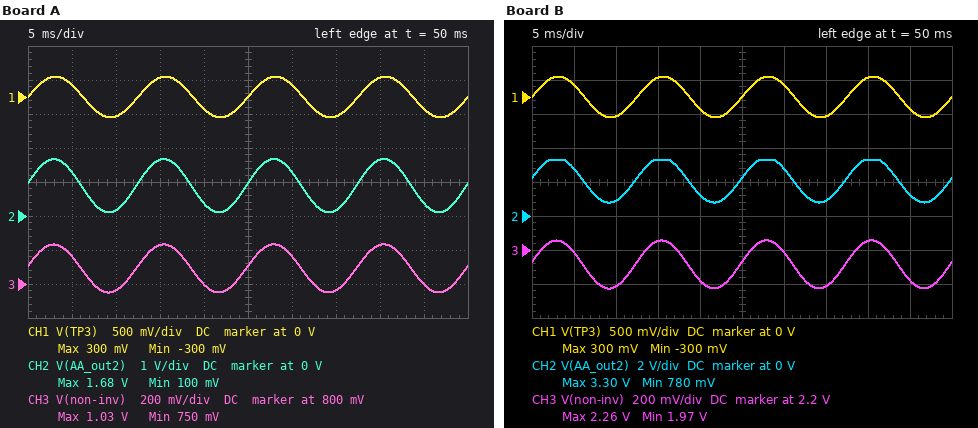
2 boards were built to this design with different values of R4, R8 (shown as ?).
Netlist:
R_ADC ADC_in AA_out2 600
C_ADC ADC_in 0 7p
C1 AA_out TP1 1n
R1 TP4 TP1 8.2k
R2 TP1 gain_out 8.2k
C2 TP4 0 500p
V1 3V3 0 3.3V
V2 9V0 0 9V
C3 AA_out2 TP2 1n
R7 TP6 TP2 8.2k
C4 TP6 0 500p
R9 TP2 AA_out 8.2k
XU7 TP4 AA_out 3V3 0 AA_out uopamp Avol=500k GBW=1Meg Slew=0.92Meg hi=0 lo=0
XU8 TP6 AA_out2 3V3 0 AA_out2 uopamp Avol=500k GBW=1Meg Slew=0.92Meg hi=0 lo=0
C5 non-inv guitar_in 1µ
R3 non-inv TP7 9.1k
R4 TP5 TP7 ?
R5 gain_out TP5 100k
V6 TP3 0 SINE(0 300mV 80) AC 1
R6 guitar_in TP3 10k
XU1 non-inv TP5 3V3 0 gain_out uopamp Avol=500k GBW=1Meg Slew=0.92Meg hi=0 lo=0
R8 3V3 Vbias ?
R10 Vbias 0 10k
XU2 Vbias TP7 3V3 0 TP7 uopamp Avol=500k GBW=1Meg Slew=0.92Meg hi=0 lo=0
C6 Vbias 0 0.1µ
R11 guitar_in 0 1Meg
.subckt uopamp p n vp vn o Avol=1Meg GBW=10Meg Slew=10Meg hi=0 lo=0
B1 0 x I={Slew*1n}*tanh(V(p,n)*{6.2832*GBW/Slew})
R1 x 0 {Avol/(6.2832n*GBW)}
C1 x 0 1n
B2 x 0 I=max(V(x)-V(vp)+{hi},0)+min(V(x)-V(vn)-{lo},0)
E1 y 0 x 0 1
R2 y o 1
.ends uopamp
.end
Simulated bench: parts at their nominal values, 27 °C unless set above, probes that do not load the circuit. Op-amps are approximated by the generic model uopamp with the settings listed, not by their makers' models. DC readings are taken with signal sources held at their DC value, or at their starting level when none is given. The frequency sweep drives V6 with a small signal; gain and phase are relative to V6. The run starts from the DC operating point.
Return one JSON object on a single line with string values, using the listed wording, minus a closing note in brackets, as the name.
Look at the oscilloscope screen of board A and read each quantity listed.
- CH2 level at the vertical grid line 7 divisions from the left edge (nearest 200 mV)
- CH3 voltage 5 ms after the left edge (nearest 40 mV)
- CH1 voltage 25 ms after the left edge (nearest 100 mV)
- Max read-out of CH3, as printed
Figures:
{"CH2 level at the vertical grid line 7 divisions from the left edge": "200 mV", "CH3 voltage 5 ms after the left edge": "960 mV", "CH1 voltage 25 ms after the left edge": "0 V", "Max read-out of CH3, as printed": "1.03 V"}
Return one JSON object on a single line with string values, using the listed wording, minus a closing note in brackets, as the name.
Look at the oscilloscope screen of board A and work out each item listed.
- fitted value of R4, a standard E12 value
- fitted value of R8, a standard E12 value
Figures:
{"fitted value of R4, a standard E12 value": "22 kΩ", "fitted value of R8, a standard E12 value": "27 kΩ"}
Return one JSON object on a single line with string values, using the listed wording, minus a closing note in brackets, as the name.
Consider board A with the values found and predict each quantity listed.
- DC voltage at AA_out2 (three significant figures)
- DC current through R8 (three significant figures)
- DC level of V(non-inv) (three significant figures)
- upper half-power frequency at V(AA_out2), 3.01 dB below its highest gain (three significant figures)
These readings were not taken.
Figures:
{"DC voltage at AA_out2": "892 mV", "DC current through R8": "89.2 µA", "DC level of V(non-inv)": "892 mV", "upper half-power frequency at V(AA_out2), 3.01 dB below its highest gain": "22.1 kHz"}
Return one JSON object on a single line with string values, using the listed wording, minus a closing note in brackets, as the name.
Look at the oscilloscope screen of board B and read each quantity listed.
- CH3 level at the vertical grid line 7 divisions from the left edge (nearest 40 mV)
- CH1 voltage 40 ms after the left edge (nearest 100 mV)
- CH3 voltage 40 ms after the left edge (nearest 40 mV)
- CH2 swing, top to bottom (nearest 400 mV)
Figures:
{"CH3 level at the vertical grid line 7 divisions from the left edge": "2.00 V", "CH1 voltage 40 ms after the left edge": "300 mV", "CH3 voltage 40 ms after the left edge": "2.24 V", "CH2 swing, top to bottom": "2.4 V"}
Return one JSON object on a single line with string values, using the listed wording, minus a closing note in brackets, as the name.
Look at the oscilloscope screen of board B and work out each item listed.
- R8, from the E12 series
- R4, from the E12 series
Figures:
{"R8, from the E12 series": "5.6 kΩ", "R4, from the E12 series": "12 kΩ"}
